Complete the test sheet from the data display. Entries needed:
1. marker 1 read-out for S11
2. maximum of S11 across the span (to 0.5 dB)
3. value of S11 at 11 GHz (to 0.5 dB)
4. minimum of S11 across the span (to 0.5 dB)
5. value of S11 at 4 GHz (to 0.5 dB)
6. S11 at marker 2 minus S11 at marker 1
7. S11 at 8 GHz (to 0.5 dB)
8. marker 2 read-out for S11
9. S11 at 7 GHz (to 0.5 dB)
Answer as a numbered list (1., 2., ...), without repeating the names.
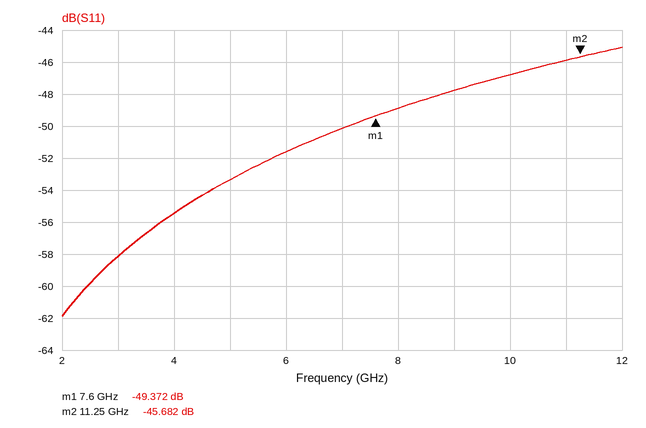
1. -49.372 dB
2. -45.0 dB
3. -46.0 dB
4. -62.0 dB
5. -55.5 dB
6. 3.690 dB
7. -49.0 dB
8. -45.682 dB
9. -50.0 dB
